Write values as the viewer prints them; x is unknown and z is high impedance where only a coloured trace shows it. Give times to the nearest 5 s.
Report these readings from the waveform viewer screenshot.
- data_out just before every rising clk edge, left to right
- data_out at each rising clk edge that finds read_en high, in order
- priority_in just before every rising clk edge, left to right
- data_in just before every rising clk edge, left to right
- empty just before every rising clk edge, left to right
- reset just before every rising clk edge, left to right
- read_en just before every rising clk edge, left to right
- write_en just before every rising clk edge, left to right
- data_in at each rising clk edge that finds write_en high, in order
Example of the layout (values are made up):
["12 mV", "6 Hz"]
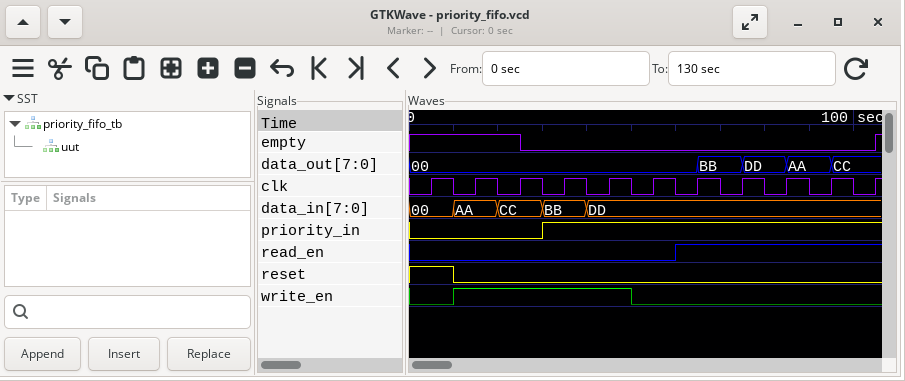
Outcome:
["00, 00, 00, 00, 00, 00, 00, BB, DD, AA, CC", "00, BB, DD, AA, CC", "0 0 0 1 1 1 1 1 1 1 1", "00, AA, CC, BB, DD, DD, DD, DD, DD, DD, DD", "1 1 1 0 0 0 0 0 0 0 0", "1 0 0 0 0 0 0 0 0 0 0", "0 0 0 0 0 0 1 1 1 1 1", "0 1 1 1 1 0 0 0 0 0 0", "AA, CC, BB, DD"]
